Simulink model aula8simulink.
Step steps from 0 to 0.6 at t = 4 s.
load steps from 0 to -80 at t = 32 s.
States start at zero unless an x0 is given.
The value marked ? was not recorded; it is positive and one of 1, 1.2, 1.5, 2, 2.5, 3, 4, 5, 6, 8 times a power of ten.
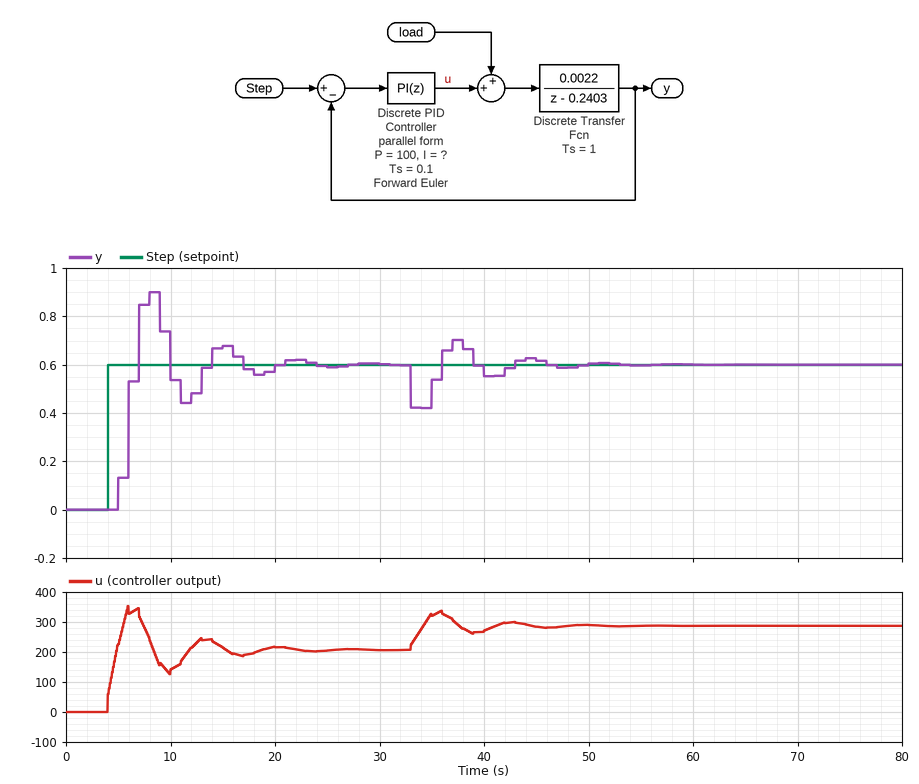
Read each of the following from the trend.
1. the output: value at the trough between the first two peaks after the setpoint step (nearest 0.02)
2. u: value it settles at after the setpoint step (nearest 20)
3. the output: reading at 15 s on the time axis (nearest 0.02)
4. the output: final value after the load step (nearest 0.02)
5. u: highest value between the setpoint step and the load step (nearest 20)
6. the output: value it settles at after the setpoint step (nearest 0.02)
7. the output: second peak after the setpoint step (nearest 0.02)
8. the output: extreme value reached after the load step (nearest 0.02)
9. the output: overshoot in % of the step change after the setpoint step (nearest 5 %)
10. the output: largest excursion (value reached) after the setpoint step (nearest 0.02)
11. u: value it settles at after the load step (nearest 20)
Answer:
0.44
200
0.68
0.60
360
0.60
0.68
0.42
50 %
0.90
280
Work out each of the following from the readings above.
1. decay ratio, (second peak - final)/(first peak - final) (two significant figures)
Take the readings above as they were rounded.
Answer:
0.27
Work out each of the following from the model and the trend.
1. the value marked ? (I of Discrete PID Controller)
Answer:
300
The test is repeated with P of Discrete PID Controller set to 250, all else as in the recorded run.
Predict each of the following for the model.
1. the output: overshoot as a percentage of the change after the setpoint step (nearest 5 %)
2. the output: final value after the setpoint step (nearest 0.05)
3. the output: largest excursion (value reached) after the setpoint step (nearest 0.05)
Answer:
20 %
0.60
0.70
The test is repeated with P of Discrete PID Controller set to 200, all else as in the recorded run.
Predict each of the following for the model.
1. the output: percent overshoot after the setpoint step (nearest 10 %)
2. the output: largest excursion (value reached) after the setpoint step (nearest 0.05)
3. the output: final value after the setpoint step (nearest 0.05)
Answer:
30 %
0.75
0.60
